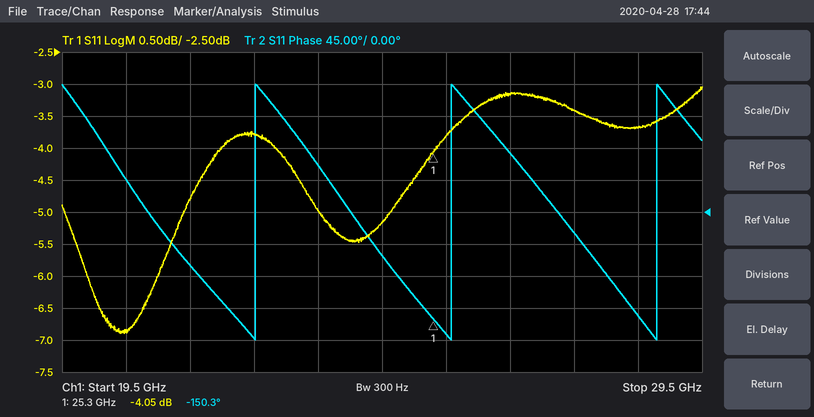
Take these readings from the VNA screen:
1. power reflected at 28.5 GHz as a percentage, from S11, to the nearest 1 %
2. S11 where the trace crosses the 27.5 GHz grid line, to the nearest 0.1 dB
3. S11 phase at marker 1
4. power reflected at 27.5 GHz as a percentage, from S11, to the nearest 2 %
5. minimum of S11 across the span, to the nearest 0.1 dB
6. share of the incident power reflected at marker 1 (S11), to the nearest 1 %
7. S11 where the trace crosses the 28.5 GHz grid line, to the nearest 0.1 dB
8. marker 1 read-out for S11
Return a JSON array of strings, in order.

["43 %", "-3.4 dB", "-150.3°", "46 %", "-6.9 dB", "39 %", "-3.7 dB", "-4.05 dB"]
